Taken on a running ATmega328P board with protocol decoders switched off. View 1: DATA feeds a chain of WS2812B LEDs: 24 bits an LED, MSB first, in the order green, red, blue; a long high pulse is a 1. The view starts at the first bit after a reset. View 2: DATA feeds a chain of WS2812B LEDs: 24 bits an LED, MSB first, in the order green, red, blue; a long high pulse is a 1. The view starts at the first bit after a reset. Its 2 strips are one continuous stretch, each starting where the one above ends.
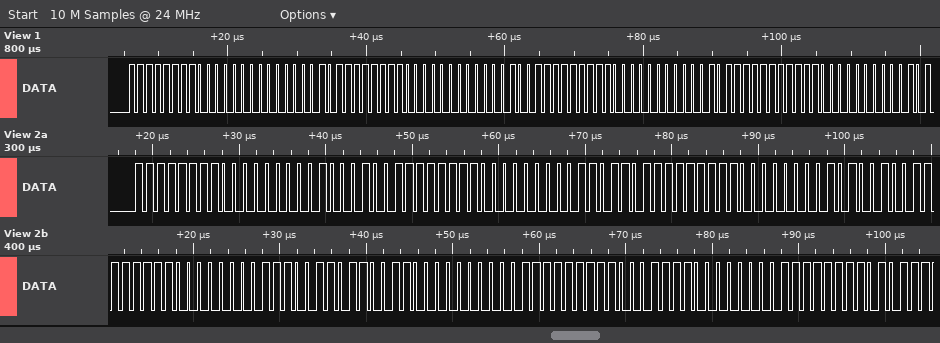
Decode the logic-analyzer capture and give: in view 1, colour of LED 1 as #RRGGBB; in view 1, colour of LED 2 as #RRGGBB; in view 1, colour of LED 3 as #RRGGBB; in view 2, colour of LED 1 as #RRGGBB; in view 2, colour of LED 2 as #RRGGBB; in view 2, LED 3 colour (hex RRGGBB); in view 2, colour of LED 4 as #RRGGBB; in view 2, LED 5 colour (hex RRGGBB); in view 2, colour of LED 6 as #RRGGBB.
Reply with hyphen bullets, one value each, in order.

- #00FF02
- #00FF09
- #00FF17
- #00FF44
- #00FF6D
- #00FFA4
- #00FFE6
- #00CCFF
- #008FFF
